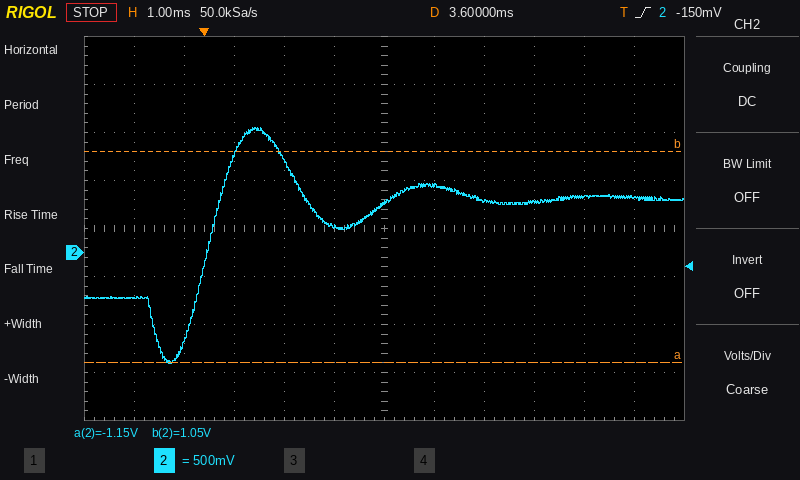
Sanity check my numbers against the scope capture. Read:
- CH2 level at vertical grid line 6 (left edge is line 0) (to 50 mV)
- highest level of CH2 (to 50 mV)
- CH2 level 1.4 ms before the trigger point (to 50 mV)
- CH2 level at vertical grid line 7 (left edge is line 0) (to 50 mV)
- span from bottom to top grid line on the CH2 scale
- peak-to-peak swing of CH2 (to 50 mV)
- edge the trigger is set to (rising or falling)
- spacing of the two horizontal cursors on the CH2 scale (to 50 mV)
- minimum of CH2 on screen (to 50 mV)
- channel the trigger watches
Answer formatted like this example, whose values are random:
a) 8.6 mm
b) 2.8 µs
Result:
a) 500 mV
b) 1.30 V
c) -450 mV
d) 700 mV
e) 4 V
f) 2.45 V
g) rising
h) 2.20 V
i) -1.15 V
j) CH2
